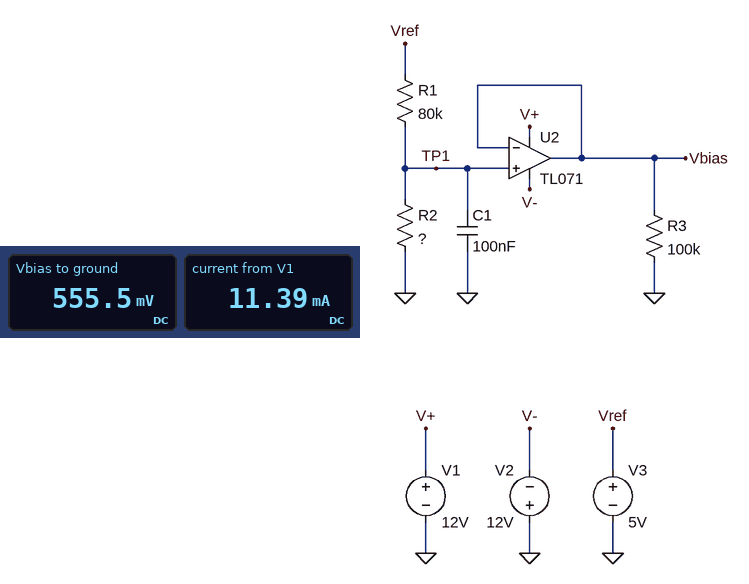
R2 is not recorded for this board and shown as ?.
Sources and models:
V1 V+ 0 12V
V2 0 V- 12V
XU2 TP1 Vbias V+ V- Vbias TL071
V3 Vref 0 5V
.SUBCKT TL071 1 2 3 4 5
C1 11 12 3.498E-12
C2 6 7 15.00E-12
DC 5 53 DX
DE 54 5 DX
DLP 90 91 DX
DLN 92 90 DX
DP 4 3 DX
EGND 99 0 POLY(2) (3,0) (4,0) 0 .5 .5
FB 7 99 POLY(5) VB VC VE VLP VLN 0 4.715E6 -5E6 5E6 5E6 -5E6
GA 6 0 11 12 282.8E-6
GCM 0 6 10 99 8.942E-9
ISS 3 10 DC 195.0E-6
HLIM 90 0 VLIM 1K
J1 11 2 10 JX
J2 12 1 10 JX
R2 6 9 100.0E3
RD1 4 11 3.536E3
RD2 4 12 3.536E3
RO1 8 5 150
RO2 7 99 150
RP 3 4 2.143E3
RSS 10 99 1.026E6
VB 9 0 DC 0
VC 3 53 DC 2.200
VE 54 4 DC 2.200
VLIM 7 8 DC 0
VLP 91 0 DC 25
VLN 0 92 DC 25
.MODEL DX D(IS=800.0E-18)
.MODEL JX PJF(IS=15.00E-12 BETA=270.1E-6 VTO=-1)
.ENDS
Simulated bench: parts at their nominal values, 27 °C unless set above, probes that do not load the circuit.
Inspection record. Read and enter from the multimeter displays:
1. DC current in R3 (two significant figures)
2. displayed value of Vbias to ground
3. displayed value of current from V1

5.6 µA
555.5 mV
11.39 mA
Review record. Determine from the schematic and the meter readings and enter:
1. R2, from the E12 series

10 kΩ
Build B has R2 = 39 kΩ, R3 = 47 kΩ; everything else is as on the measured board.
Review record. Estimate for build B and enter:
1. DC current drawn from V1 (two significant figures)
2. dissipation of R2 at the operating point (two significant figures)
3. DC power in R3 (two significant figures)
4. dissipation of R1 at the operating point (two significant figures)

11 mA
69 µW
57 µW
140 µW
